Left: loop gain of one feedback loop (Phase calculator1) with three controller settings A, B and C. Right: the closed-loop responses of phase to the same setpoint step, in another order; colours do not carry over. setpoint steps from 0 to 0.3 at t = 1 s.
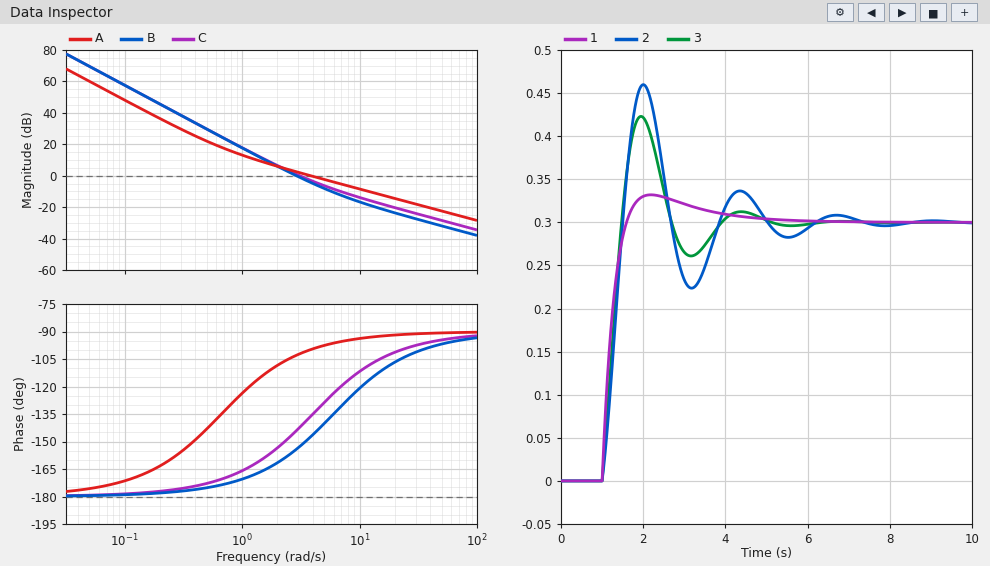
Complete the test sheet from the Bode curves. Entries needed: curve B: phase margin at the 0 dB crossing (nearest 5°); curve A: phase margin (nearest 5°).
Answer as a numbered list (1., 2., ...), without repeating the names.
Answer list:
1. 25°
2. 80°
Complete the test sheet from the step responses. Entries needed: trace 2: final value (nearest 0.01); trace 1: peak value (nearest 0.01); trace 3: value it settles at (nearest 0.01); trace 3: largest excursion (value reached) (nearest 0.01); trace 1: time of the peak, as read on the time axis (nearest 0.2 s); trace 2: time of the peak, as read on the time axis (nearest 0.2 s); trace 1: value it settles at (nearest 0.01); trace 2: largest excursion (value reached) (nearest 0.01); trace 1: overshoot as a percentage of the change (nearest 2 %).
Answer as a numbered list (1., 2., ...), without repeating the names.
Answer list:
1. 0.30
2. 0.33
3. 0.30
4. 0.42
5. 2.2 s
6. 2.0 s
7. 0.30
8. 0.46
9. 10 %
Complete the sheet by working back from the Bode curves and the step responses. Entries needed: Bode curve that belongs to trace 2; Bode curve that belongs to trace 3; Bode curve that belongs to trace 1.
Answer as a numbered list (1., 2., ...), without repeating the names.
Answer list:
1. B
2. C
3. A
